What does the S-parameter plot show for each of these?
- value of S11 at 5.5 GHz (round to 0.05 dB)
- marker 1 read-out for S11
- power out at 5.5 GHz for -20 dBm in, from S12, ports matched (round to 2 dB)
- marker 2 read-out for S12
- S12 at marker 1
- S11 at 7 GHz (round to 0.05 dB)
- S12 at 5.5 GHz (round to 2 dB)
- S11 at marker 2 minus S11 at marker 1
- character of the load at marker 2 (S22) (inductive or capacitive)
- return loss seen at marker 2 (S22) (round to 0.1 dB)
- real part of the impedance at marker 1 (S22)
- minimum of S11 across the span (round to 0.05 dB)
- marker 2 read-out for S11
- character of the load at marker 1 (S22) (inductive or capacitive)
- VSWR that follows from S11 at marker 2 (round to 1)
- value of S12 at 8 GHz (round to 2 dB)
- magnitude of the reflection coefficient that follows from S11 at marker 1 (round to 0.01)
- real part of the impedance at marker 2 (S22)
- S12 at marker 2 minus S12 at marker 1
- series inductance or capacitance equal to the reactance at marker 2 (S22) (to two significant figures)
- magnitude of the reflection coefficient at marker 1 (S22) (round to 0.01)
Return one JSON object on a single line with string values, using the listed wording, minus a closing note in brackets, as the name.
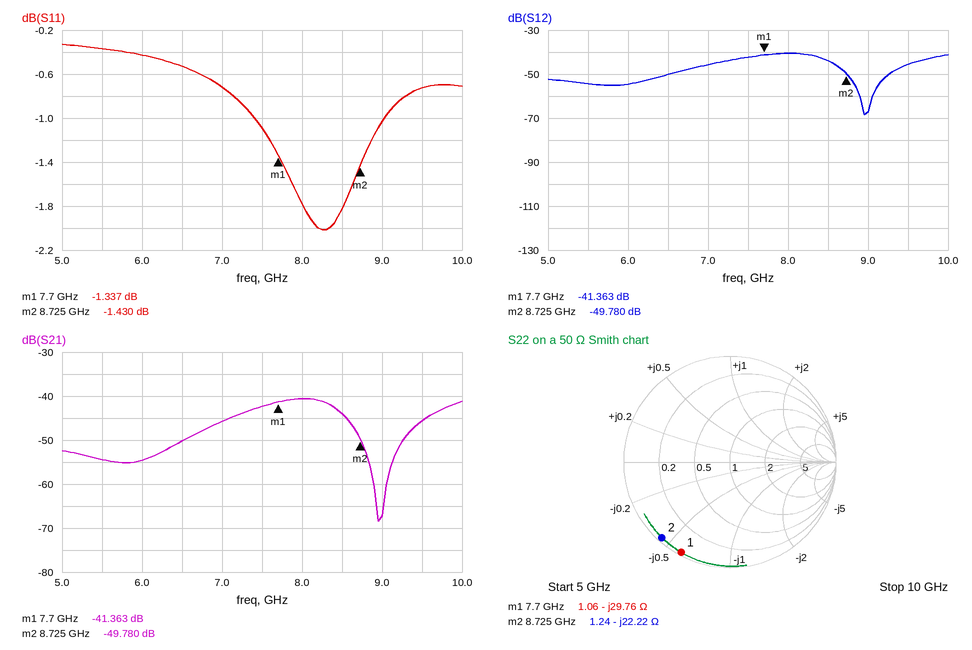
{"value of S11 at 5.5 GHz": "-0.35 dB", "marker 1 read-out for S11": "-1.337 dB", "power out at 5.5 GHz for -20 dBm in, from S12, ports matched": "-74 dBm", "marker 2 read-out for S12": "-49.780 dB", "S12 at marker 1": "-41.363 dB", "S11 at 7 GHz": "-0.70 dB", "S12 at 5.5 GHz": "-54 dB", "S11 at marker 2 minus S11 at marker 1": "-0.093 dB", "character of the load at marker 2 (S22)": "capacitive", "return loss seen at marker 2 (S22)": "0.4 dB", "real part of the impedance at marker 1": "1.06 Ω", "minimum of S11 across the span": "-2.00 dB", "marker 2 read-out for S11": "-1.430 dB", "character of the load at marker 1 (S22)": "capacitive", "VSWR that follows from S11 at marker 2": "12", "value of S12 at 8 GHz": "-40 dB", "magnitude of the reflection coefficient that follows from S11 at marker 1": "0.86", "real part of the impedance at marker 2": "1.24 Ω", "S12 at marker 2 minus S12 at marker 1": "-8.417 dB", "series inductance or capacitance equal to the reactance at marker 2 (S22)": "820 fF", "magnitude of the reflection coefficient at marker 1 (S22)": "0.97"}
